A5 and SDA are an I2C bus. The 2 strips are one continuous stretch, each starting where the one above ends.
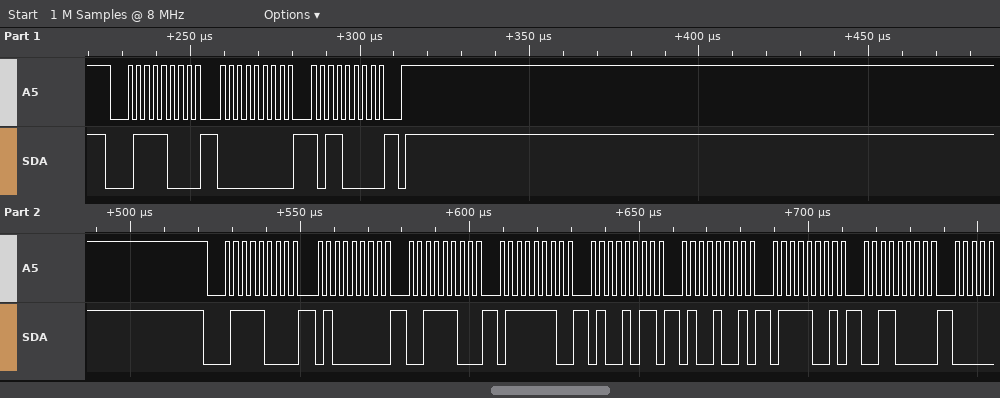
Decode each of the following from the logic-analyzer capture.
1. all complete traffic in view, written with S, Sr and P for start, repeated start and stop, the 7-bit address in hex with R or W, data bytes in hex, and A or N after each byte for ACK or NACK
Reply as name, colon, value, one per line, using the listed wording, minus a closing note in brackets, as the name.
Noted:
all complete traffic in view, written with S, Sr and P for start, repeated start and stop, the 7-bit address in hex with R or W, data bytes in hex, and A or N after each byte for ACK or NACK: S 3CW A 00 A B0 A P S 3CW A 40 A 3C A 7E A 4B A 49 A 79 A 30 A
